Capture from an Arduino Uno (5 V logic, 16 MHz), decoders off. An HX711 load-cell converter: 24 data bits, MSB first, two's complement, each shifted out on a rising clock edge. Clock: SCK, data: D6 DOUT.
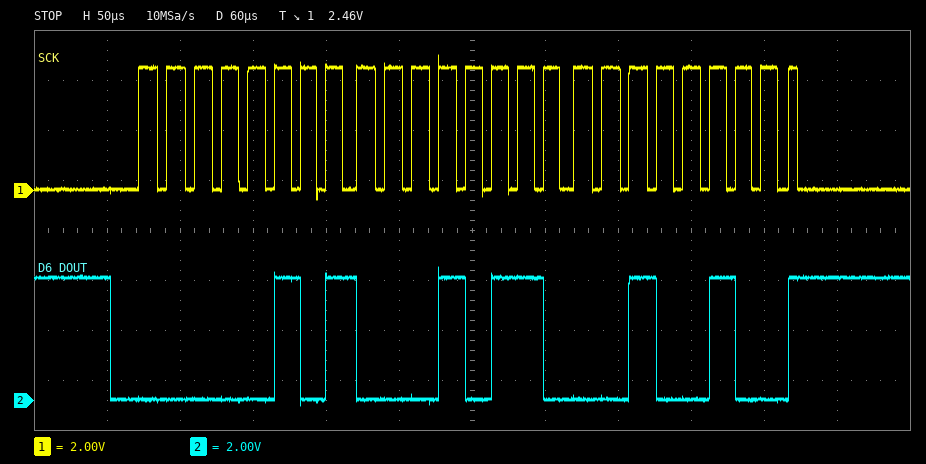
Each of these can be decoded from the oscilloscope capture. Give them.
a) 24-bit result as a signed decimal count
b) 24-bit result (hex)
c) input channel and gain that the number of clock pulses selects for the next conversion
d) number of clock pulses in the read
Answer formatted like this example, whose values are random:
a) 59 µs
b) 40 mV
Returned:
a) 333348
b) 0x051624
c) channel A, gain 128
d) 25
